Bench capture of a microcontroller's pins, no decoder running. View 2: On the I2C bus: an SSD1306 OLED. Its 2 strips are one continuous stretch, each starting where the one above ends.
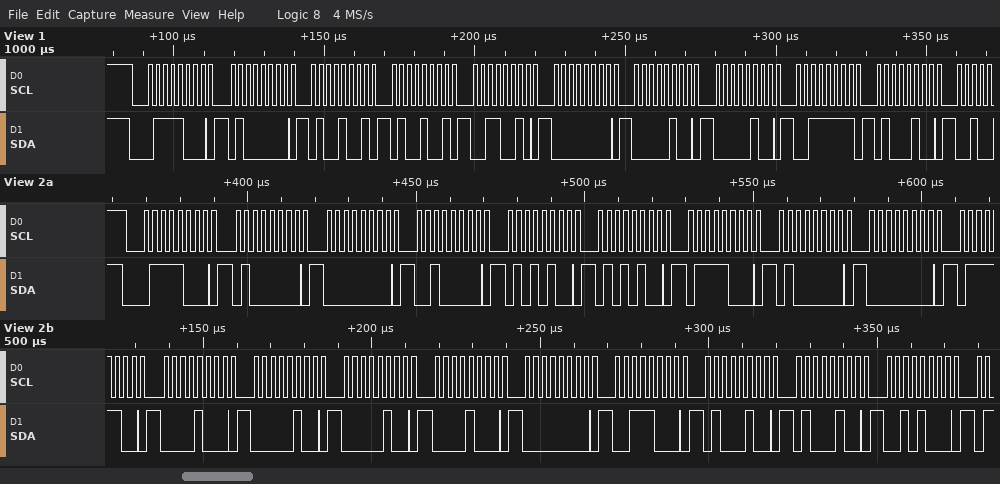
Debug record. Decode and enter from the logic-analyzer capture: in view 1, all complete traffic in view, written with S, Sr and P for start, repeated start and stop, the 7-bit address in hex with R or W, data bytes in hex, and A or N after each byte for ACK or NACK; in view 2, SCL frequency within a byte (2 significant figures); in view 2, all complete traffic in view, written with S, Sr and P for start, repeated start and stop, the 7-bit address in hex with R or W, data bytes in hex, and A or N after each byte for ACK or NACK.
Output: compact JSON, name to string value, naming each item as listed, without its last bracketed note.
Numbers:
{"in view 1, all complete traffic in view, written with S, Sr and P for start, repeated start and stop, the 7-bit address in hex with R or W, data bytes in hex, and A or N after each byte for ACK or NACK": "S 3CW A 40 A 49 A 49 A 32 A 00 A 04 A 04 A 3F A 44 A", "in view 2, SCL frequency within a byte": "400 kHz", "in view 2, all complete traffic in view, written with S, Sr and P for start, repeated start and stop, the 7-bit address in hex with R or W, data bytes in hex, and A or N after each byte for ACK or NACK": "S 3CW A 40 A 00 A 20 A 54 A 54 A 78 A 40 A 00 A 7C A 08 A 04 A 04 A 08 A 00 A 38 A 44 A 44 A 28 A"}
